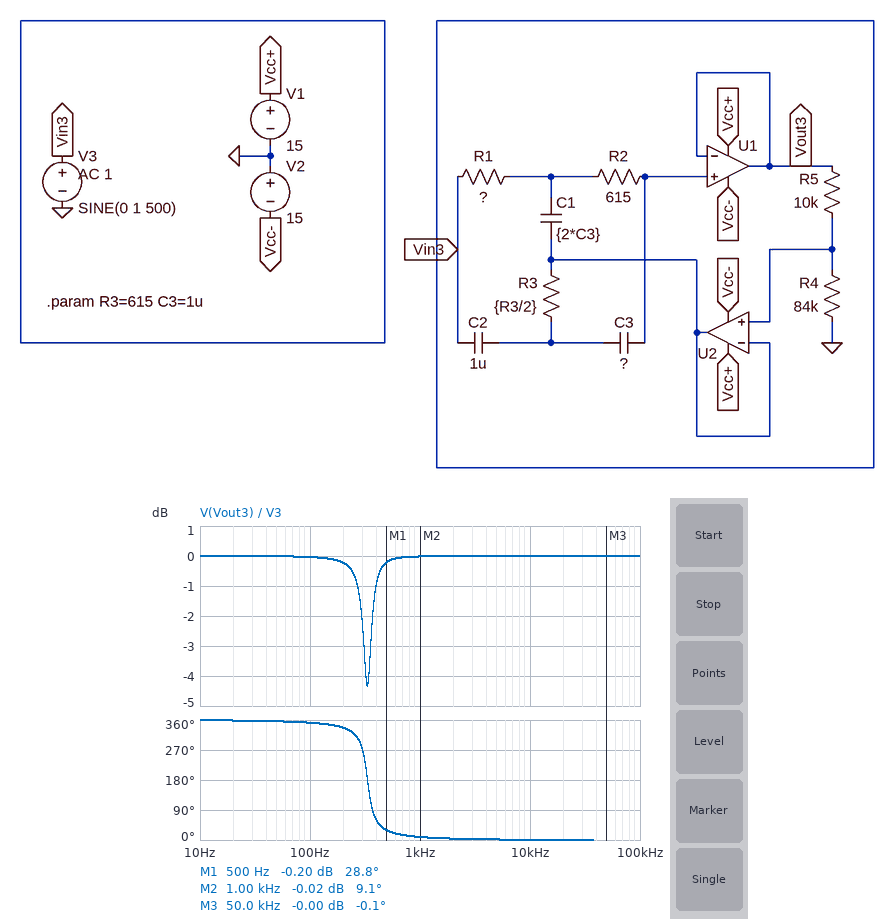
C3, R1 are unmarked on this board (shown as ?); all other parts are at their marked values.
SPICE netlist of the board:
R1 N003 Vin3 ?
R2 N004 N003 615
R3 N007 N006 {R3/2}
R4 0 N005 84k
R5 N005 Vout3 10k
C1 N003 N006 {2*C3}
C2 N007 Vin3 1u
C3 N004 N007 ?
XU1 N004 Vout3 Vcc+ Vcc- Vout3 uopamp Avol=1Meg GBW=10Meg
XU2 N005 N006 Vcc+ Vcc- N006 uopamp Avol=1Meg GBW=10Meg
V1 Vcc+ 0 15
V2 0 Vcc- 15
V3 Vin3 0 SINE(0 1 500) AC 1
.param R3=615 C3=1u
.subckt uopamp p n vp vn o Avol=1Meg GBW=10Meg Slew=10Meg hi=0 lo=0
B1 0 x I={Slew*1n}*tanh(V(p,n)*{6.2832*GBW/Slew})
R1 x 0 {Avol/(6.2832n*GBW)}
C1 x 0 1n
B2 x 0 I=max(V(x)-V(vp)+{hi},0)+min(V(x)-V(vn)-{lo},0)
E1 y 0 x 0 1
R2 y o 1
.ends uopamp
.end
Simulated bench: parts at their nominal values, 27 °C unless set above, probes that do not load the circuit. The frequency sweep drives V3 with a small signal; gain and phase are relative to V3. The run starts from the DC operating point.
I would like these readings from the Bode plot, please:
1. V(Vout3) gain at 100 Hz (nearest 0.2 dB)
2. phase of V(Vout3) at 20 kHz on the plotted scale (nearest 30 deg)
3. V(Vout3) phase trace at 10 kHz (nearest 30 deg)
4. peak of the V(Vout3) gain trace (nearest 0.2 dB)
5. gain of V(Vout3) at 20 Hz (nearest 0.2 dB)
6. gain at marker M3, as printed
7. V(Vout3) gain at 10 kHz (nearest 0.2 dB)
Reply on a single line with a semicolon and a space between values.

0 dB; 0 deg; 0 deg; 0 dB; 0 dB; -0.00 dB; 0 dB
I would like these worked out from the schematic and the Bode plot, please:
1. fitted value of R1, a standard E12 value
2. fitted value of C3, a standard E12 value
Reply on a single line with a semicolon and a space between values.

680 Ω; 470 nF
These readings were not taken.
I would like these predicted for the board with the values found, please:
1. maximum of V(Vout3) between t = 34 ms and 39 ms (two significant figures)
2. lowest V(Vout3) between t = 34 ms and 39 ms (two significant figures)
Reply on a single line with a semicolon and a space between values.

980 mV; -980 mV
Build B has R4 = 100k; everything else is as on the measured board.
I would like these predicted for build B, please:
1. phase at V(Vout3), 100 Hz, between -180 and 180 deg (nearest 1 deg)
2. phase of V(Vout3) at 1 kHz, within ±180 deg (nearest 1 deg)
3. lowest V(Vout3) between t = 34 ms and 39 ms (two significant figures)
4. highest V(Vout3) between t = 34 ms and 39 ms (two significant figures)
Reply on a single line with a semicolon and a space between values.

-7 deg; 8 deg; -1.0 V; 1.0 V
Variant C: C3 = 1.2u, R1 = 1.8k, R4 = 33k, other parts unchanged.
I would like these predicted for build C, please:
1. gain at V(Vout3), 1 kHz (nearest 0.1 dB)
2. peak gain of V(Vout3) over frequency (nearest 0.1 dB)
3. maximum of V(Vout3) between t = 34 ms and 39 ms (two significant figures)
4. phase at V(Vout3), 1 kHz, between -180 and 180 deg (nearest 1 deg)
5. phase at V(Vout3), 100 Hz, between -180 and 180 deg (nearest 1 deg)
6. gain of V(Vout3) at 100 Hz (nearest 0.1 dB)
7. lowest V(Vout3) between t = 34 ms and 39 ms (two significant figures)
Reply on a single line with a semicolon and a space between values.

-0.2 dB; 0 dB; 910 mV; 13 deg; -62 deg; -4.8 dB; -910 mV
